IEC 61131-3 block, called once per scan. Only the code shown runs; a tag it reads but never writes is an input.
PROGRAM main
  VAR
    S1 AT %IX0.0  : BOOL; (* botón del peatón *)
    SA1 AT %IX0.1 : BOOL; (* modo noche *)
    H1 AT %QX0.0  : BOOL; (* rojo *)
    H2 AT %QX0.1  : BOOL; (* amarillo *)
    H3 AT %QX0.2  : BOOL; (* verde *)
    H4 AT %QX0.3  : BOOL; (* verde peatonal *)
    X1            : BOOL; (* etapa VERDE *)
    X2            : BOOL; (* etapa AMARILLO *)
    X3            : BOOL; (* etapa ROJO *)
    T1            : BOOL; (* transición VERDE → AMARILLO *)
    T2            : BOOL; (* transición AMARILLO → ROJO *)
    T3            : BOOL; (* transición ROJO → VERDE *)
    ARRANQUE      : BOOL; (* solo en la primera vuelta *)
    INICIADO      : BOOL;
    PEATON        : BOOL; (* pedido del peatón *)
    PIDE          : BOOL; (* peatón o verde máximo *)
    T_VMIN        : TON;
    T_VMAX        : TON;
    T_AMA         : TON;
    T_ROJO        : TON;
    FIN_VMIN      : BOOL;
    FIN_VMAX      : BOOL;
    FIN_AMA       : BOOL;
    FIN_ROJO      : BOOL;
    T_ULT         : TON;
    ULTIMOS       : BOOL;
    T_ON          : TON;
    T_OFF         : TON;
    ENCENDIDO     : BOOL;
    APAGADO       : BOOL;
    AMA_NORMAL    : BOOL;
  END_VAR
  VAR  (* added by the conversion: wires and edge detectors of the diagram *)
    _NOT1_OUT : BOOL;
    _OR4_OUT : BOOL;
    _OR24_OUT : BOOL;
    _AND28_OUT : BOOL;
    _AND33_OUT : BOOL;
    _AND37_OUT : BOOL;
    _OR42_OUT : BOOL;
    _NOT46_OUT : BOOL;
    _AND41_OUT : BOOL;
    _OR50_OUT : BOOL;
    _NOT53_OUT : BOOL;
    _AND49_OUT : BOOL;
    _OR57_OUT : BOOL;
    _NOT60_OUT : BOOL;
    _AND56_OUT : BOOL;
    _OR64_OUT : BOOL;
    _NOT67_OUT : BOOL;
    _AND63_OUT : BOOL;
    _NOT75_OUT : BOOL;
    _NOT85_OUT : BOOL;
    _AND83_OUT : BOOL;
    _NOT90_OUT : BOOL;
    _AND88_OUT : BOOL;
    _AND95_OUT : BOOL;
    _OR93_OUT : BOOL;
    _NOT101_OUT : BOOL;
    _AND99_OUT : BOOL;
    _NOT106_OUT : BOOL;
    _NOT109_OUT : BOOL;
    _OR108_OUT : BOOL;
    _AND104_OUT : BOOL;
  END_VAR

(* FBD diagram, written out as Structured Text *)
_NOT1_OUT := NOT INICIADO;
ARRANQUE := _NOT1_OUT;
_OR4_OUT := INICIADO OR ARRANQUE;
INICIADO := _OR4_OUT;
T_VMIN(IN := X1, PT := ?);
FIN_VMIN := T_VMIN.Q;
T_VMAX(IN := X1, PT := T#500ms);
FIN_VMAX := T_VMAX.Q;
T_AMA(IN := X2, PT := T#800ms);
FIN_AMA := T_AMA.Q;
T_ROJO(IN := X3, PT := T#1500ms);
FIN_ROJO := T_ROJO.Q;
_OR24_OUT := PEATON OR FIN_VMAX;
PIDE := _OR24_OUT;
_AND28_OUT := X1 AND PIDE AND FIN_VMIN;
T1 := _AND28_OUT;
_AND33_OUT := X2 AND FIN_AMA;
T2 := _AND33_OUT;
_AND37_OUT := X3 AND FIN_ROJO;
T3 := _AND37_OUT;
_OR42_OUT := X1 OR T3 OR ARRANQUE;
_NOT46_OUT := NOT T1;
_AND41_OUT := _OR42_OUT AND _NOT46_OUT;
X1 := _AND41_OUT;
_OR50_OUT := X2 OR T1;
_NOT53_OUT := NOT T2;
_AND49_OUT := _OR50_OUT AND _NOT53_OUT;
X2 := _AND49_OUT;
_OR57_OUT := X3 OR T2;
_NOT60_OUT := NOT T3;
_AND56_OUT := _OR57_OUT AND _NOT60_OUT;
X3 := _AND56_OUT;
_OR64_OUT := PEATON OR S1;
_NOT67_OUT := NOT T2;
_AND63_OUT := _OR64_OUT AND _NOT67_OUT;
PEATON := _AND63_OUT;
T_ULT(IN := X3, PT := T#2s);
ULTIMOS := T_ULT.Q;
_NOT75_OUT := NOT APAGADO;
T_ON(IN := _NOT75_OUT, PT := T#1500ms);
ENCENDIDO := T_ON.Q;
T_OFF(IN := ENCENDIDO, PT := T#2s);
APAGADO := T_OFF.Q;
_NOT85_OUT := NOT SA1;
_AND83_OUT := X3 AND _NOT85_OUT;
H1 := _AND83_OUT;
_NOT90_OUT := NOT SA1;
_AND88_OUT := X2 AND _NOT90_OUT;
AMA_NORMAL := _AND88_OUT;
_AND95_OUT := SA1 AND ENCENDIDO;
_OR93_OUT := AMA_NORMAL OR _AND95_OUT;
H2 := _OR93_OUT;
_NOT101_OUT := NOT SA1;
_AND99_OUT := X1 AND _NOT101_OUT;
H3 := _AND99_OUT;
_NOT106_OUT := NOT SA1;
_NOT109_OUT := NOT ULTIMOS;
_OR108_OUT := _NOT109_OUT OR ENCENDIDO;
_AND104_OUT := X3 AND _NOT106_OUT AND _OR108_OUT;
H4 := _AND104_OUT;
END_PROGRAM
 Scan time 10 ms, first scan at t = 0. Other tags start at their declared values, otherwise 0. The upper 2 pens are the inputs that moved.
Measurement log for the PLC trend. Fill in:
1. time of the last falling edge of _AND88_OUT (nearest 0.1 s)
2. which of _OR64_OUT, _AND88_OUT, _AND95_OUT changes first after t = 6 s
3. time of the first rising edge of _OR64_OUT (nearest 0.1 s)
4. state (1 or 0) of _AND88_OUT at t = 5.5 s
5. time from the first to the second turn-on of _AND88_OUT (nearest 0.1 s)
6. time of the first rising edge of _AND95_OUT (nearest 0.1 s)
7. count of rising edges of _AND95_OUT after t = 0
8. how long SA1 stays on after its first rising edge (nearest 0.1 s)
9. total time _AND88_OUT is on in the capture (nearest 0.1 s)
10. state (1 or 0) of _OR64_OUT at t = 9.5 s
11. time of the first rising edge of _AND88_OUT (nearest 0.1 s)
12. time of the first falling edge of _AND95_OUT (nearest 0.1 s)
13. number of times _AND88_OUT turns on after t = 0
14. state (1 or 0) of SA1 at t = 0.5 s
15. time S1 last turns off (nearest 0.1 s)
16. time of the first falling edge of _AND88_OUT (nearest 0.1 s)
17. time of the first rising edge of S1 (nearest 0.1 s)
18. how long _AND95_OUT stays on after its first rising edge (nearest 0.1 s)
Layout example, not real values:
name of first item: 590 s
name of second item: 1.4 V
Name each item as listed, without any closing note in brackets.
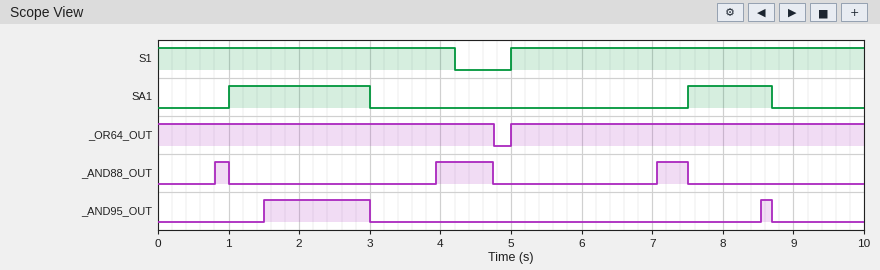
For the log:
time of the last falling edge of _AND88_OUT: 7.5 s
which of _OR64_OUT, _AND88_OUT, _AND95_OUT changes first after t = 6 s: _AND88_OUT
time of the first rising edge of _OR64_OUT: 5.0 s
state (1 or 0) of _AND88_OUT at t = 5.5 s: 0
time from the first to the second turn-on of _AND88_OUT: 3.1 s
time of the first rising edge of _AND95_OUT: 1.5 s
count of rising edges of _AND95_OUT after t = 0: 2
how long SA1 stays on after its first rising edge: 2.0 s
total time _AND88_OUT is on in the capture: 1.4 s
state (1 or 0) of _OR64_OUT at t = 9.5 s: 1
time of the first rising edge of _AND88_OUT: 0.8 s
time of the first falling edge of _AND95_OUT: 3.0 s
number of times _AND88_OUT turns on after t = 0: 3
state (1 or 0) of SA1 at t = 0.5 s: 0
time S1 last turns off: 4.2 s
time of the first falling edge of _AND88_OUT: 1.0 s
time of the first rising edge of S1: 5.0 s
how long _AND95_OUT stays on after its first rising edge: 1.5 s
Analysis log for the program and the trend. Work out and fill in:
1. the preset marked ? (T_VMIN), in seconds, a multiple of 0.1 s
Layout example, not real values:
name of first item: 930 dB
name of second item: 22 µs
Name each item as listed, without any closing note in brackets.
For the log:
the preset marked ? (T_VMIN), in seconds, a multiple of 0.1 s: 0.8 s
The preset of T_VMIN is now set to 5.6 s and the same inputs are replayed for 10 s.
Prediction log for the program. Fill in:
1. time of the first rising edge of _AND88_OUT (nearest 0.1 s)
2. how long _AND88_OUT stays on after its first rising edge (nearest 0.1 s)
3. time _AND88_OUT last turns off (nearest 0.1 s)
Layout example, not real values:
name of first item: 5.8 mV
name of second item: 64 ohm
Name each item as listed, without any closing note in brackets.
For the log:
time of the first rising edge of _AND88_OUT: 5.6 s
how long _AND88_OUT stays on after its first rising edge: 0.8 s
time _AND88_OUT last turns off: 6.4 s
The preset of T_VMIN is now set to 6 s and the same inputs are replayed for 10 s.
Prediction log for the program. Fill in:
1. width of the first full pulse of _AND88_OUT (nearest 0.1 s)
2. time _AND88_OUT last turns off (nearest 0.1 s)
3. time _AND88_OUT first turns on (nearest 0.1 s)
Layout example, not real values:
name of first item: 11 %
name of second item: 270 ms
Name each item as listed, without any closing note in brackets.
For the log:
width of the first full pulse of _AND88_OUT: 0.8 s
time _AND88_OUT last turns off: 6.8 s
time _AND88_OUT first turns on: 6.0 s
